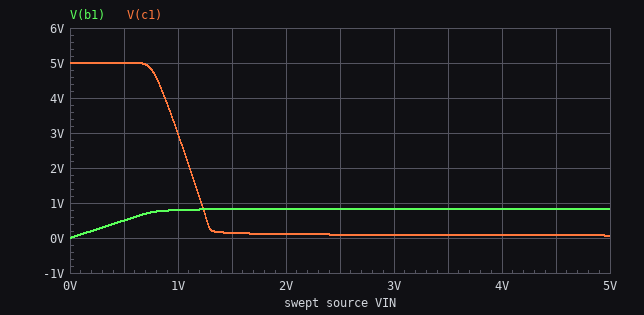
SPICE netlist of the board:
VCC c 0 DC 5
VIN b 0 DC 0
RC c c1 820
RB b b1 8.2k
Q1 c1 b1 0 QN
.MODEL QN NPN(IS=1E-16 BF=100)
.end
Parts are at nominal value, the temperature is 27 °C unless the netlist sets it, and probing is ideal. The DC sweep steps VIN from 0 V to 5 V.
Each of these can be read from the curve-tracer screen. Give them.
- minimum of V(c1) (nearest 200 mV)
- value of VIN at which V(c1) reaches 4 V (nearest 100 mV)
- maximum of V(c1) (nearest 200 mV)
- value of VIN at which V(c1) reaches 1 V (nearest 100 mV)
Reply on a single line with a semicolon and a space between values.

0 V; 900 mV; 5.0 V; 1.2 V
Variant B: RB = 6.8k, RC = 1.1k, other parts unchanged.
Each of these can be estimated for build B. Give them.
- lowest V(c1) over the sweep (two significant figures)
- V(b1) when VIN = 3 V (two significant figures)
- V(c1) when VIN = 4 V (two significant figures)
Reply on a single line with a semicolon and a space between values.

60 mV; 820 mV; 66 mV
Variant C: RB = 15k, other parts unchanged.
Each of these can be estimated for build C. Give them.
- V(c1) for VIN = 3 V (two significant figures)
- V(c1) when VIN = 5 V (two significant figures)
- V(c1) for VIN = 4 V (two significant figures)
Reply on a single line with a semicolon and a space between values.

110 mV; 88 mV; 97 mV
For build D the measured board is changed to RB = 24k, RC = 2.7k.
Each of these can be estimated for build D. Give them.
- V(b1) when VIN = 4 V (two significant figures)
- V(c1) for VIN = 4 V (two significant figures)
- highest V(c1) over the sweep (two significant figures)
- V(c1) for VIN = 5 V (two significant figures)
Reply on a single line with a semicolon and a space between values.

790 mV; 75 mV; 5.0 V; 68 mV
